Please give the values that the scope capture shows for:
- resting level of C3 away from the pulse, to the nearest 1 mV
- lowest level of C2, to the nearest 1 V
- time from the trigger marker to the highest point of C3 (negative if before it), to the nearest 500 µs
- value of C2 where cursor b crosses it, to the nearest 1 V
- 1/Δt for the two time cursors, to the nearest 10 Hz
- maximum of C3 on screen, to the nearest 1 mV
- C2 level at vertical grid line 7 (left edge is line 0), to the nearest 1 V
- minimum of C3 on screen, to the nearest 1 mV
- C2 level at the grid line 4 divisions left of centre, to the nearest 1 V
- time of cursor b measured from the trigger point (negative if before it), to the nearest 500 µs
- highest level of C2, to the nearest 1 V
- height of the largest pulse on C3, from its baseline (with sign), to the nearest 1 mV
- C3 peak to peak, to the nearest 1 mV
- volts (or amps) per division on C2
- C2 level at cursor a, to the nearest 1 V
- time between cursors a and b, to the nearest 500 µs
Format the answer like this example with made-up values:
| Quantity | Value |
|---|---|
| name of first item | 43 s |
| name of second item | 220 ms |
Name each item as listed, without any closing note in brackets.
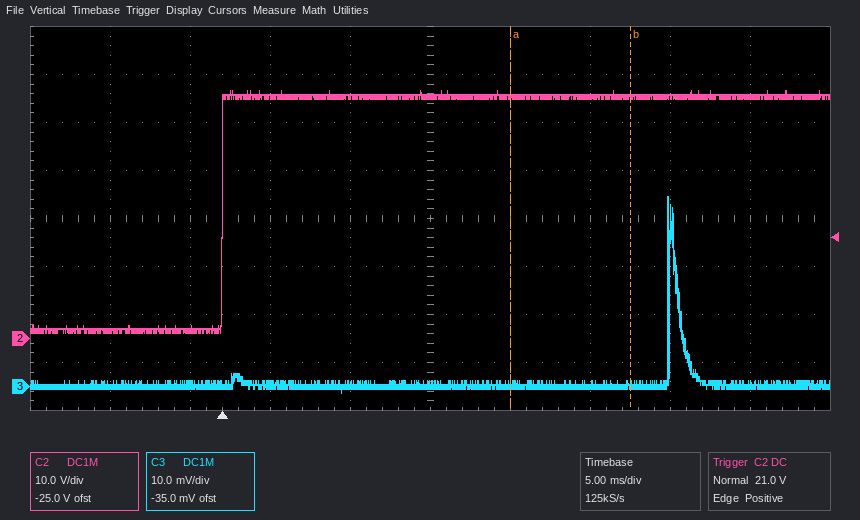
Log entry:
| Quantity | Value |
|---|---|
| resting level of C3 away from the pulse, to the nearest 1 mV | 0 mV |
| lowest level of C2, to the nearest 1 V | 1 V |
| time from the trigger marker to the highest point of C3 (negative if before it), to the nearest 500 µs | +28.0 ms |
| value of C2 where cursor b crosses it, to the nearest 1 V | 50 V |
| 1/Δt for the two time cursors, to the nearest 10 Hz | 130 Hz |
| maximum of C3 on screen, to the nearest 1 mV | 40 mV |
| C2 level at vertical grid line 7 (left edge is line 0), to the nearest 1 V | 50 V |
| minimum of C3 on screen, to the nearest 1 mV | -1 mV |
| C2 level at the grid line 4 divisions left of centre, to the nearest 1 V | 2 V |
| time of cursor b measured from the trigger point (negative if before it), to the nearest 500 µs | +25.5 ms |
| highest level of C2, to the nearest 1 V | 52 V |
| height of the largest pulse on C3, from its baseline (with sign), to the nearest 1 mV | +40 mV |
| C3 peak to peak, to the nearest 1 mV | 41 mV |
| volts (or amps) per division on C2 | 10 V |
| C2 level at cursor a, to the nearest 1 V | 50 V |
| time between cursors a and b, to the nearest 500 µs | 7.5 ms |
